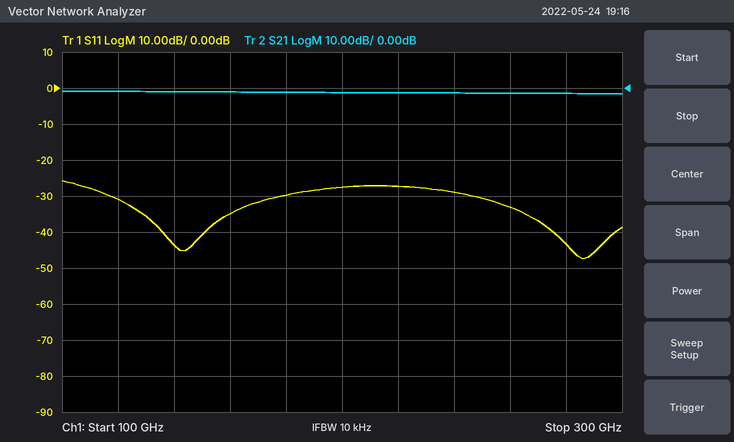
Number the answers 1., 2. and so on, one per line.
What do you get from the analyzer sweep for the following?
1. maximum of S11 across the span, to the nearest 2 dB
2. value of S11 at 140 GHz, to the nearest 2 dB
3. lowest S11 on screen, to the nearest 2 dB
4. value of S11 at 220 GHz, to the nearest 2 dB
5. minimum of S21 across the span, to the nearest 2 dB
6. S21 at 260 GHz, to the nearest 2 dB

1. -26 dB
2. -44 dB
3. -48 dB
4. -28 dB
5. -2 dB
6. -2 dB
